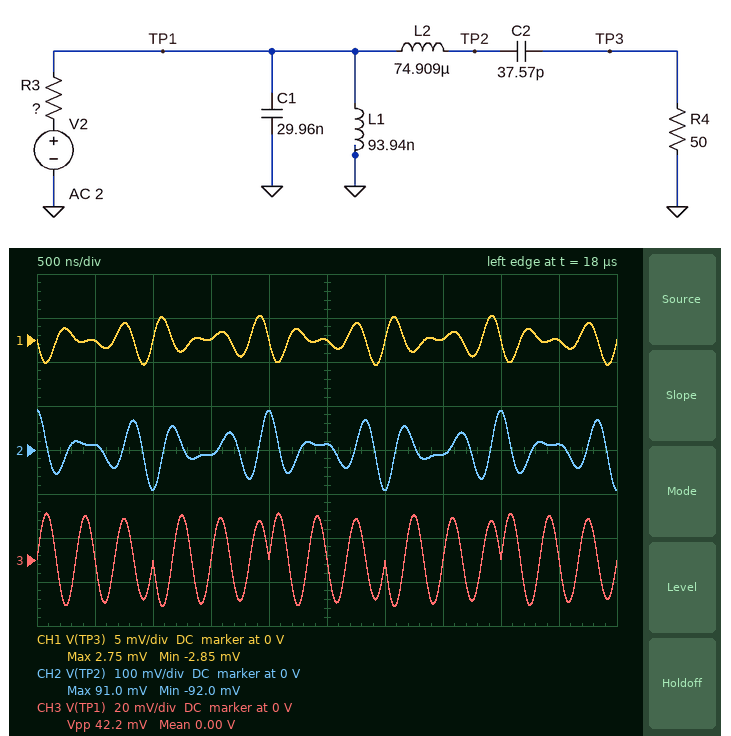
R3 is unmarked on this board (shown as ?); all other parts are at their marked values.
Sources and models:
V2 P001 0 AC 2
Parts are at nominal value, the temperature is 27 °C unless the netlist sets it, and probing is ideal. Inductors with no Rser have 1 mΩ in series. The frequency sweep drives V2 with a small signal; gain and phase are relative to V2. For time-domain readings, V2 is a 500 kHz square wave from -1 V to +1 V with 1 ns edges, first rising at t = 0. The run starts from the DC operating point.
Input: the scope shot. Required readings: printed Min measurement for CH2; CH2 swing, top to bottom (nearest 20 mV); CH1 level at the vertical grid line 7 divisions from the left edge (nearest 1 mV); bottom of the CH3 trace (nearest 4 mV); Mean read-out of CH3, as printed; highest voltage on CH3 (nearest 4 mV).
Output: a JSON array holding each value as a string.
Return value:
["-92.0 mV", "180 mV", "0 V", "-20 mV", "0.00 V", "20 mV"]
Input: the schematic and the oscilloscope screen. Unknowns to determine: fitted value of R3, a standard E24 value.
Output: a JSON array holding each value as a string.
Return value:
["91 Ω"]
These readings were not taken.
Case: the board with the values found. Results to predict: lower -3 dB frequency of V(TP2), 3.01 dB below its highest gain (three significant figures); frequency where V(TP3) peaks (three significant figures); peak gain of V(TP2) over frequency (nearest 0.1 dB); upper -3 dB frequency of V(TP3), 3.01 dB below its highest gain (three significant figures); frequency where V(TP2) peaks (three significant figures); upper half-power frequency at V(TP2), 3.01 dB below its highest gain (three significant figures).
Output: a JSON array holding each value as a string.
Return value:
["2.93 MHz", "2.97 MHz", "20.2 dB", "3.07 MHz", "2.97 MHz", "3.07 MHz"]
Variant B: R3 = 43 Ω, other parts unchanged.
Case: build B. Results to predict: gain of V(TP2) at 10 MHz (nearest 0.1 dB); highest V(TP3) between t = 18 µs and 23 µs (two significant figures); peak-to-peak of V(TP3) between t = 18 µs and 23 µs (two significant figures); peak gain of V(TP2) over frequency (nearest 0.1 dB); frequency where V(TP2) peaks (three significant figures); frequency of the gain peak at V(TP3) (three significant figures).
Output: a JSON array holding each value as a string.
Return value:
["-57.4 dB", "5.9 mV", "12 mV", "23.6 dB", "2.99 MHz", "3.00 MHz"]
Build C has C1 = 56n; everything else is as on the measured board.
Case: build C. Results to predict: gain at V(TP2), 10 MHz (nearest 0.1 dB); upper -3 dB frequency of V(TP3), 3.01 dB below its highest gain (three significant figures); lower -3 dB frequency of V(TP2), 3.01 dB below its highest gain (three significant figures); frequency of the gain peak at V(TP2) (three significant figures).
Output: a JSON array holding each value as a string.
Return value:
["-69.7 dB", "2.21 MHz", "2.18 MHz", "2.19 MHz"]
